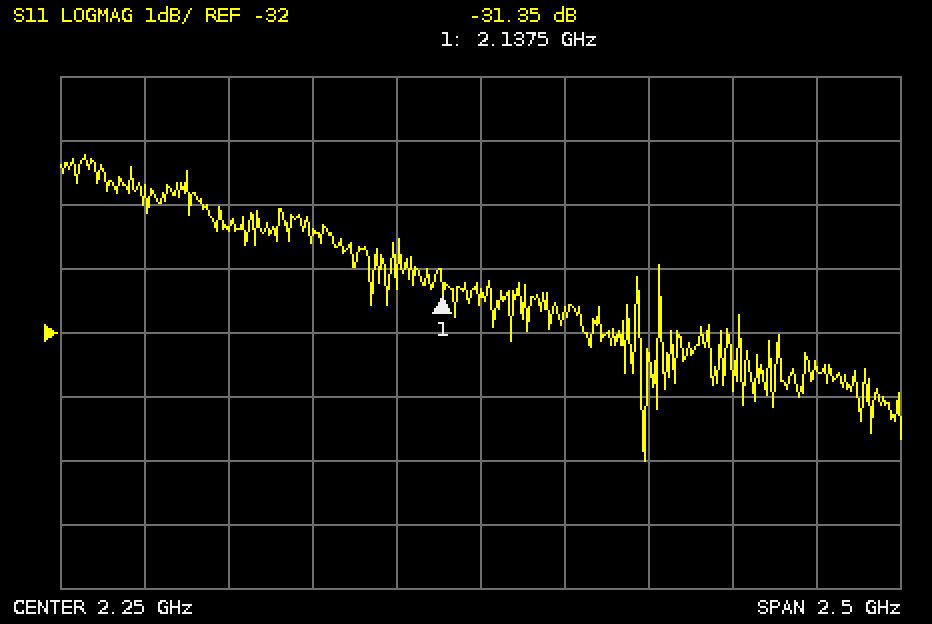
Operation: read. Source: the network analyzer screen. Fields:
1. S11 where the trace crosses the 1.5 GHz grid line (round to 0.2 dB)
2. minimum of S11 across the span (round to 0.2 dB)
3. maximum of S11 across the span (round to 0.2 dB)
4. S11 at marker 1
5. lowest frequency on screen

-30.4 dB
-34.0 dB
-29.2 dB
-31.35 dB
1 GHz
